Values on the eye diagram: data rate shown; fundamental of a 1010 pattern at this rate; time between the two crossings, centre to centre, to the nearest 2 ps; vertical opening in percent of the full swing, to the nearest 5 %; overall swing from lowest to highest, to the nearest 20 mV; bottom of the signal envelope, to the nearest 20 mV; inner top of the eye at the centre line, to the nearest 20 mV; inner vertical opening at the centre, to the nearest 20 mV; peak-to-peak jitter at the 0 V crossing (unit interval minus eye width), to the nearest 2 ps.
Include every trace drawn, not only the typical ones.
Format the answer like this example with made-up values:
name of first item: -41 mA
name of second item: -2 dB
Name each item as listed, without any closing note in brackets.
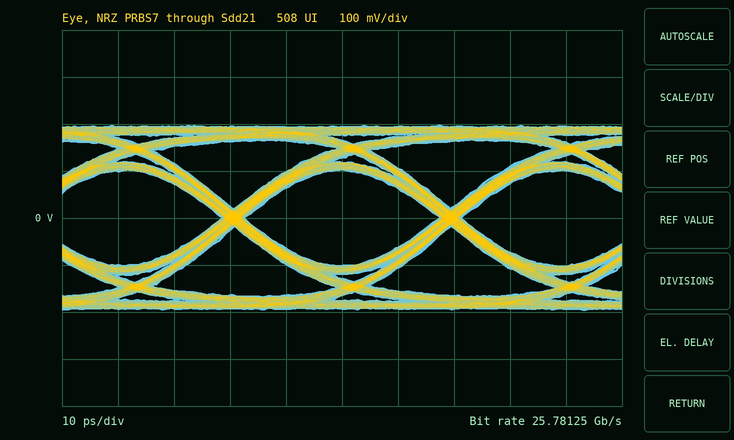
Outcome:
data rate shown: 25.78125 Gb/s
fundamental of a 1010 pattern at this rate: 12.89062 GHz
time between the two crossings, centre to centre, to the nearest 2 ps: 38 ps
vertical opening in percent of the full swing, to the nearest 5 %: 50 %
overall swing from lowest to highest, to the nearest 20 mV: 400 mV
bottom of the signal envelope, to the nearest 20 mV: -200 mV
inner top of the eye at the centre line, to the nearest 20 mV: 100 mV
inner vertical opening at the centre, to the nearest 20 mV: 200 mV
peak-to-peak jitter at the 0 V crossing (unit interval minus eye width), to the nearest 2 ps: 4 ps
